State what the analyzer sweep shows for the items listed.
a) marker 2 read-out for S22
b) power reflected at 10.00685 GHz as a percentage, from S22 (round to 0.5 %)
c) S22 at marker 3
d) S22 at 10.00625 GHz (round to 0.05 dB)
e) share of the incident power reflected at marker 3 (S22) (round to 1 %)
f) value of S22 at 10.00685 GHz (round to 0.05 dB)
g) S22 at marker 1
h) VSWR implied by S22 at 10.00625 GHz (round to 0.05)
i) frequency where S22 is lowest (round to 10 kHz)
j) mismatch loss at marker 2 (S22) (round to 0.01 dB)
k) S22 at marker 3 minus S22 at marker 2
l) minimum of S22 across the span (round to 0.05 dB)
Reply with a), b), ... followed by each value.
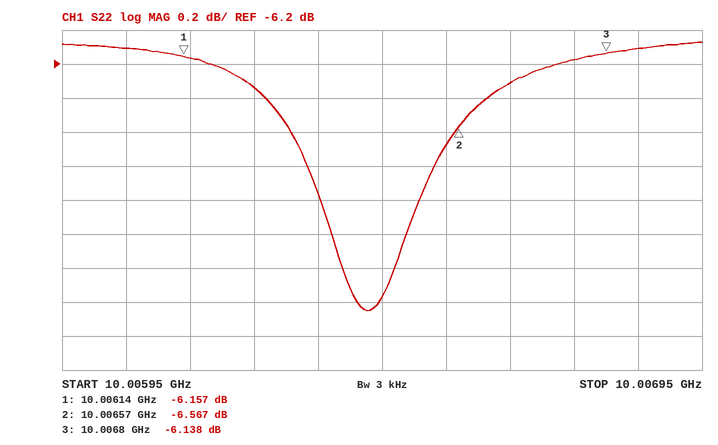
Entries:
a) -6.567 dB
b) 24.5 %
c) -6.138 dB
d) -6.35 dB
e) 24 %
f) -6.10 dB
g) -6.157 dB
h) 2.85
i) 10.00643 GHz
j) 1.08 dB
k) 0.429 dB
l) -7.65 dB
